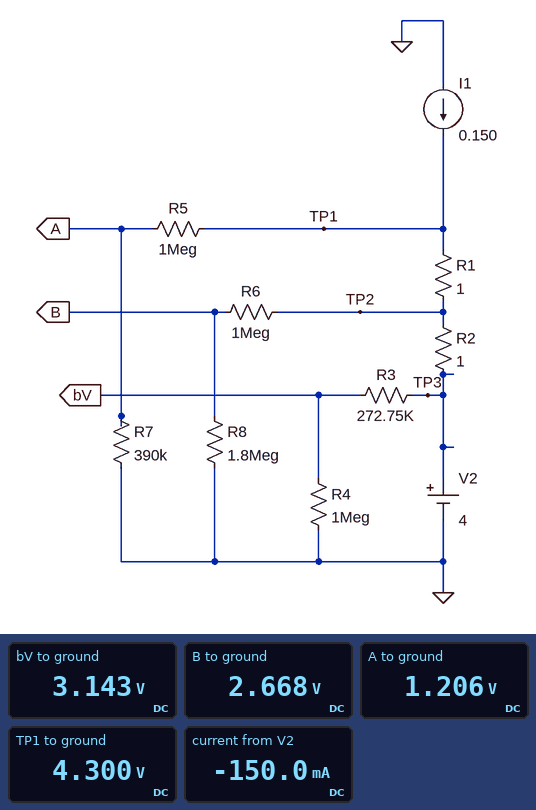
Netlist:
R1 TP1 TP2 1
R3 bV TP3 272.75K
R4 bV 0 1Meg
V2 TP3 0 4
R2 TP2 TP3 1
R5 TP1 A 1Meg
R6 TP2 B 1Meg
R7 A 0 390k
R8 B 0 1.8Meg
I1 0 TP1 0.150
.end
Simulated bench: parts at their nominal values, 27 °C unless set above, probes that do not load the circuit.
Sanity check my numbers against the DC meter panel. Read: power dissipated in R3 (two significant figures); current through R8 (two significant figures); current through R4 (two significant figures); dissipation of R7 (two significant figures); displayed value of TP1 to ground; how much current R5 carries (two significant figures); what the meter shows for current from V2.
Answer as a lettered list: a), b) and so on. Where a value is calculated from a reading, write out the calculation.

a) (4 V - 3.143 V)^2 / 272.8 kΩ = 2.7 µW
b) (2.668 V) / 1.8 MΩ = 1.5 µA
c) (3.143 V) / 1 MΩ = 3.1 µA
d) (1.206 V)^2 / 390 kΩ = 3.7 µW
e) 4.300 V
f) (4.3 V - 1.206 V) / 1 MΩ = 3.1 µA
g) -150.0 mA
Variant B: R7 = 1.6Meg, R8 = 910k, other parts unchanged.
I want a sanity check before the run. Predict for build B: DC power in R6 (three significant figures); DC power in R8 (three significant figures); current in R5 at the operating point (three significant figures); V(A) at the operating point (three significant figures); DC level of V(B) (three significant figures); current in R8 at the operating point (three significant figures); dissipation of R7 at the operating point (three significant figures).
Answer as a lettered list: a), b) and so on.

a) 4.72 µW
b) 4.30 µW
c) 1.65 µA
d) 2.65 V
e) 1.98 V
f) 2.17 µA
g) 4.38 µW
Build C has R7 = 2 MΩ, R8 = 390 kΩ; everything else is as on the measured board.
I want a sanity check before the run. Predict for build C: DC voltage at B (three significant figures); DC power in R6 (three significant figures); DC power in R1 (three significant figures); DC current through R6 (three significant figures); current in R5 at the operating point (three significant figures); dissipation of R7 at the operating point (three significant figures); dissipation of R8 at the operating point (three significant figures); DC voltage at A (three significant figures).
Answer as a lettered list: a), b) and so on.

a) 1.16 V
b) 8.91 µW
c) 22.5 mW
d) 2.99 µA
e) 1.43 µA
f) 4.11 µW
g) 3.48 µW
h) 2.87 V
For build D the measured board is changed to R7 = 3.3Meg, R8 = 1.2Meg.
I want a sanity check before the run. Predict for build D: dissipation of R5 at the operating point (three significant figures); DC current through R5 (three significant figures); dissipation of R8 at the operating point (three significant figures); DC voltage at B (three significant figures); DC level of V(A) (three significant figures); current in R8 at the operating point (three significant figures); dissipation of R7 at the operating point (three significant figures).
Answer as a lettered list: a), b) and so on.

a) 1.00 µW
b) 1.00 µA
c) 4.27 µW
d) 2.26 V
e) 3.30 V
f) 1.89 µA
g) 3.30 µW
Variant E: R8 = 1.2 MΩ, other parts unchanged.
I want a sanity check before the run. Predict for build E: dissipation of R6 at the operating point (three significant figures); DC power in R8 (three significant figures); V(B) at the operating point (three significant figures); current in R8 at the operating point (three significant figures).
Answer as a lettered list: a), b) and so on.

a) 3.56 µW
b) 4.27 µW
c) 2.26 V
d) 1.89 µA
